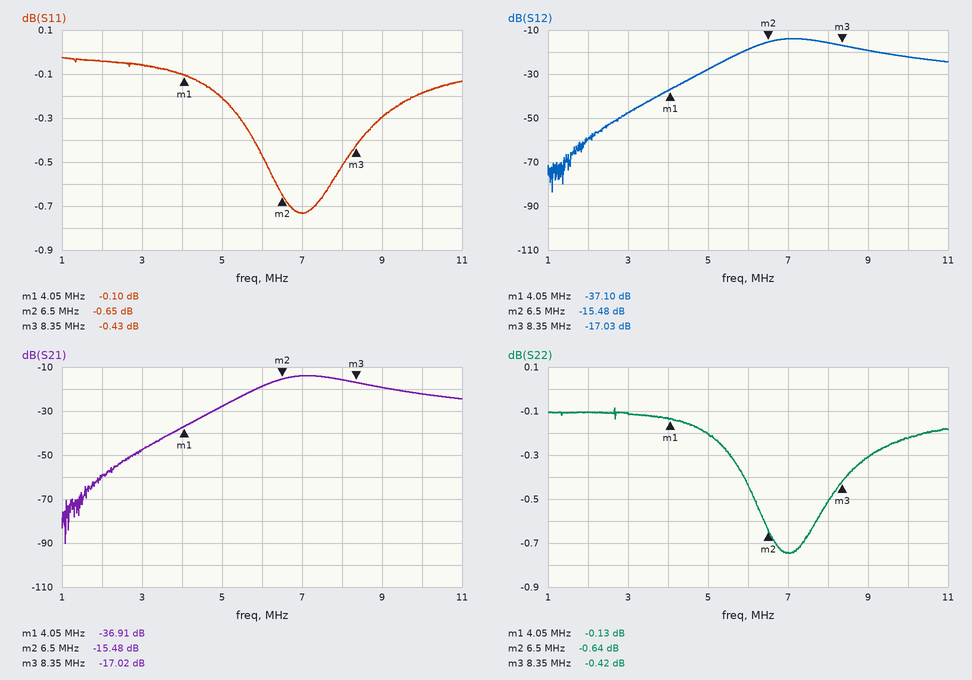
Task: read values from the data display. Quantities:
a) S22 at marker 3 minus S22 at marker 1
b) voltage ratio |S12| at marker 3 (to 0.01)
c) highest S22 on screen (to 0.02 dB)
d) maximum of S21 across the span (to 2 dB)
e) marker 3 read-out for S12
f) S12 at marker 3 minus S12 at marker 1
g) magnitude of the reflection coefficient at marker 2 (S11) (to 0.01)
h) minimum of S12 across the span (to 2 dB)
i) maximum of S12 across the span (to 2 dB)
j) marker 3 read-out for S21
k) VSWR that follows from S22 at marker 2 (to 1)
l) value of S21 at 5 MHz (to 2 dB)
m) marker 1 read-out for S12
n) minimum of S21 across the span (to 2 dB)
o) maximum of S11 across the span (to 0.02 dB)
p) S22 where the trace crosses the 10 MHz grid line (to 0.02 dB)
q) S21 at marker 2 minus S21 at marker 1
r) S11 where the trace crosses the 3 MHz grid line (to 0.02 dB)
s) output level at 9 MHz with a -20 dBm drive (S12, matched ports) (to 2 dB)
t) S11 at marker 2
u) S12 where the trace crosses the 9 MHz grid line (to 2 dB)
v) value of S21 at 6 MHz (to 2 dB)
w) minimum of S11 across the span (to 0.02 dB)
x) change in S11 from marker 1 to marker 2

-0.29 dB
0.14
-0.08 dB
-14 dB
-17.03 dB
20.07 dB
0.93
-84 dB
-14 dB
-17.02 dB
27
-28 dB
-37.10 dB
-90 dB
-0.02 dB
-0.22 dB
21.43 dB
-0.06 dB
-40 dBm
-0.65 dB
-20 dB
-18 dB
-0.74 dB
-0.55 dB
